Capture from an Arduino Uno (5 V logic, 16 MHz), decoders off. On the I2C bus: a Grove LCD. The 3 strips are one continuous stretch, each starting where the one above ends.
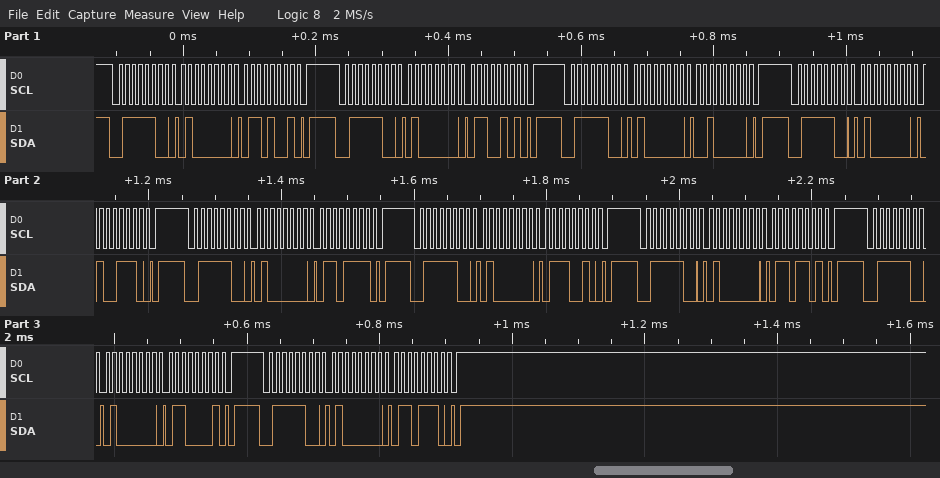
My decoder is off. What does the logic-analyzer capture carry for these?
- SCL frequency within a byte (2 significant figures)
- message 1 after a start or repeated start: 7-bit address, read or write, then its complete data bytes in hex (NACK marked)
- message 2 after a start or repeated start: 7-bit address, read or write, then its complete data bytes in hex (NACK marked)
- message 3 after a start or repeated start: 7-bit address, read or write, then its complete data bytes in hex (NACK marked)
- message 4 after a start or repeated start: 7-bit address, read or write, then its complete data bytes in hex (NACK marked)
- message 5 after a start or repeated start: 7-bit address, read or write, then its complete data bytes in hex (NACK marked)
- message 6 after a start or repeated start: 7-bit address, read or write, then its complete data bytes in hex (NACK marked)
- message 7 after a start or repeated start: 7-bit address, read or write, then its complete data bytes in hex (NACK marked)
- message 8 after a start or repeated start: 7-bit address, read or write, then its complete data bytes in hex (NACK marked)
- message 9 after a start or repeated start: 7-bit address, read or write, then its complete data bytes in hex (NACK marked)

100 kHz
0x3E write: 40 69
0x3E write: 40 65
0x3E write: 40 20
0x3E write: 40 4E
0x3E write: 40 6F
0x3E write: 40 72
0x3E write: 40 6D
0x3E write: 40 61
0x3E write: 40 6E
